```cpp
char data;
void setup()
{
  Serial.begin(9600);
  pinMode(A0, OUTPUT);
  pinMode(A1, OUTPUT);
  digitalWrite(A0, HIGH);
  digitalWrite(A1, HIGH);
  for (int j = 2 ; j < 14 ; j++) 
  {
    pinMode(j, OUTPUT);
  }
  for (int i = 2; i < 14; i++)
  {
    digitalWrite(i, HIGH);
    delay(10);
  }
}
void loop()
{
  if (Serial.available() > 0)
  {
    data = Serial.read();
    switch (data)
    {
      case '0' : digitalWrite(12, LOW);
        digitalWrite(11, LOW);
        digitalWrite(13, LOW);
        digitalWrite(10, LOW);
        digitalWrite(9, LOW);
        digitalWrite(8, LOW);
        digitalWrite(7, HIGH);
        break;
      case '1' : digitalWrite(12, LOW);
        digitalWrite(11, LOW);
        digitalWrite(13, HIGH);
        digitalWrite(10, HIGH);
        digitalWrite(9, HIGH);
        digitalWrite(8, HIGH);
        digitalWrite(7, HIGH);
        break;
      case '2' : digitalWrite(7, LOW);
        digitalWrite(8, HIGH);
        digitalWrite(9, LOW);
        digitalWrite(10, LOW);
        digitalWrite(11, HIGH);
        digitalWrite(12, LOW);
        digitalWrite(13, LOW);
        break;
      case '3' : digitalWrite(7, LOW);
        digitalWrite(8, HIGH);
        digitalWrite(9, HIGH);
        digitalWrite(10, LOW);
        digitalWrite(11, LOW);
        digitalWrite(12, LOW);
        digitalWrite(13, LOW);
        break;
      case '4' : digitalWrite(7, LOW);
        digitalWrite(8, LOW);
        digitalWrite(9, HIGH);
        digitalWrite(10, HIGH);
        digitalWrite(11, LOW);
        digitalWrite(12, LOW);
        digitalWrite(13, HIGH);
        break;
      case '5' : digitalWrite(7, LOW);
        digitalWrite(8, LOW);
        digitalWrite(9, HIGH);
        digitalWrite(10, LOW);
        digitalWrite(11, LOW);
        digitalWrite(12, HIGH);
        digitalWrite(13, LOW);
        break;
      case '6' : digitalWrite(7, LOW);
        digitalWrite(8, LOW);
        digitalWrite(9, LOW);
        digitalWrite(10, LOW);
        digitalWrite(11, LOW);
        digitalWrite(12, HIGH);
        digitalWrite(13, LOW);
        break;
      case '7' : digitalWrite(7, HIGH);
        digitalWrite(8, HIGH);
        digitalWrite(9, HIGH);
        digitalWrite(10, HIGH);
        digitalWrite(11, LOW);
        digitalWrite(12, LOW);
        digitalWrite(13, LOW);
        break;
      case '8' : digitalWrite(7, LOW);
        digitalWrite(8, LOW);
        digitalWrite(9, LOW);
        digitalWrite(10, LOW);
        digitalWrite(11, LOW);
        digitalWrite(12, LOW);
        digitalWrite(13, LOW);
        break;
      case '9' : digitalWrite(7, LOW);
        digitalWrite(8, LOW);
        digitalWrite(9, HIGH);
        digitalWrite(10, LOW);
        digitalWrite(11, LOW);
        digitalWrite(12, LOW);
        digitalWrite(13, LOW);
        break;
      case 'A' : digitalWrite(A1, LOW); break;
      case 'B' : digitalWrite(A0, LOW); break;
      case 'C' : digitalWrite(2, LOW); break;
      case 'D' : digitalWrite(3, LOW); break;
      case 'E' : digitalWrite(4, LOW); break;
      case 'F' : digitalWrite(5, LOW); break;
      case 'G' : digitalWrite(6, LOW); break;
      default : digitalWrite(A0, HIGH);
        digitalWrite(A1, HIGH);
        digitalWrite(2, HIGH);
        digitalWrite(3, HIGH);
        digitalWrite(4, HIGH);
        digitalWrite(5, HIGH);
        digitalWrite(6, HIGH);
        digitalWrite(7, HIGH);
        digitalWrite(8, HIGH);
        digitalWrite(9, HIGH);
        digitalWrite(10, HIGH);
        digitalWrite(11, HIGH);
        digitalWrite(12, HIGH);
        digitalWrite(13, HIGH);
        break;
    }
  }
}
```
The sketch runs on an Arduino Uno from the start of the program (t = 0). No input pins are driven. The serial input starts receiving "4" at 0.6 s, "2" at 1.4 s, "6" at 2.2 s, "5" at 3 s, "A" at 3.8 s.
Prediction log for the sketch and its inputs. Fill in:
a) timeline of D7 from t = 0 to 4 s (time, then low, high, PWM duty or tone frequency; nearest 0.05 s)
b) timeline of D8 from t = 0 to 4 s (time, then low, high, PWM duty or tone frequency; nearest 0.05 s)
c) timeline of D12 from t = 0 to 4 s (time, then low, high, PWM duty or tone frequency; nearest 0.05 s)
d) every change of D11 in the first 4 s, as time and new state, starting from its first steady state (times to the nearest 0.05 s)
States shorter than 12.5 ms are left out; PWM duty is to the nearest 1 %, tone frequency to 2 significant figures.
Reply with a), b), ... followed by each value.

a) 0 s low; 0.05 s high; 0.6 s low
b) 0 s low; 0.05 s high; 0.6 s low; 1.4 s high; 2.2 s low
c) 0 s low; 0.1 s high; 0.6 s low; 2.2 s high
d) 0 s low; 0.1 s high; 0.6 s low; 1.4 s high; 2.2 s low
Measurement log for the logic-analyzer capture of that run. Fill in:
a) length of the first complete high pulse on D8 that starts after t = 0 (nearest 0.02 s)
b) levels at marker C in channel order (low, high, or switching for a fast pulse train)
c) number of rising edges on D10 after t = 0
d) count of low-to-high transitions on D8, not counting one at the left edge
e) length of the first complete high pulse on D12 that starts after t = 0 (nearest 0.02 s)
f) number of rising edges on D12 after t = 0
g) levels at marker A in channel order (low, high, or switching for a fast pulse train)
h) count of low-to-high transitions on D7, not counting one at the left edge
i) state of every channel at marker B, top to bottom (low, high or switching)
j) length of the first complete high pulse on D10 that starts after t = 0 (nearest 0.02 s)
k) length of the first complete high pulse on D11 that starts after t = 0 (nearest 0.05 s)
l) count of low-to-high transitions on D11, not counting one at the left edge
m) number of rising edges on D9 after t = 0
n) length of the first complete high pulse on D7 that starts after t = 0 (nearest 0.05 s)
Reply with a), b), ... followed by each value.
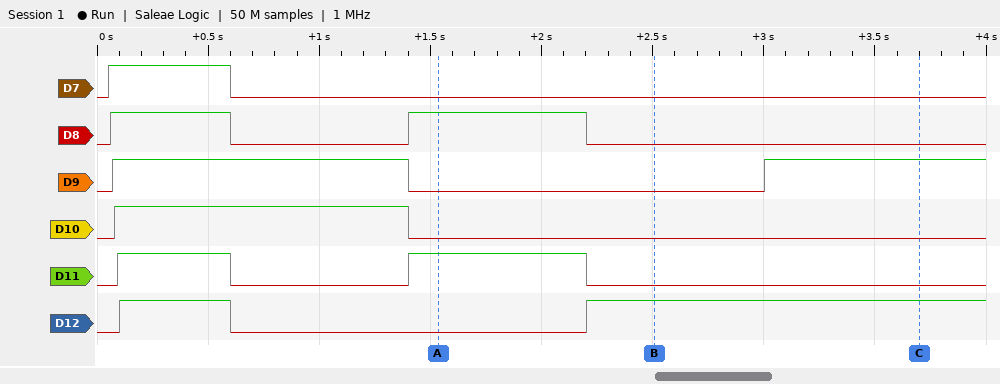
a) 0.54 s
b) D7 low, D8 low, D9 high, D10 low, D11 low, D12 high
c) 1
d) 2
e) 0.50 s
f) 2
g) D7 low, D8 high, D9 low, D10 low, D11 high, D12 low
h) 1
i) D7 low, D8 low, D9 low, D10 low, D11 low, D12 high
j) 1.32 s
k) 0.50 s
l) 2
m) 2
n) 0.55 s
